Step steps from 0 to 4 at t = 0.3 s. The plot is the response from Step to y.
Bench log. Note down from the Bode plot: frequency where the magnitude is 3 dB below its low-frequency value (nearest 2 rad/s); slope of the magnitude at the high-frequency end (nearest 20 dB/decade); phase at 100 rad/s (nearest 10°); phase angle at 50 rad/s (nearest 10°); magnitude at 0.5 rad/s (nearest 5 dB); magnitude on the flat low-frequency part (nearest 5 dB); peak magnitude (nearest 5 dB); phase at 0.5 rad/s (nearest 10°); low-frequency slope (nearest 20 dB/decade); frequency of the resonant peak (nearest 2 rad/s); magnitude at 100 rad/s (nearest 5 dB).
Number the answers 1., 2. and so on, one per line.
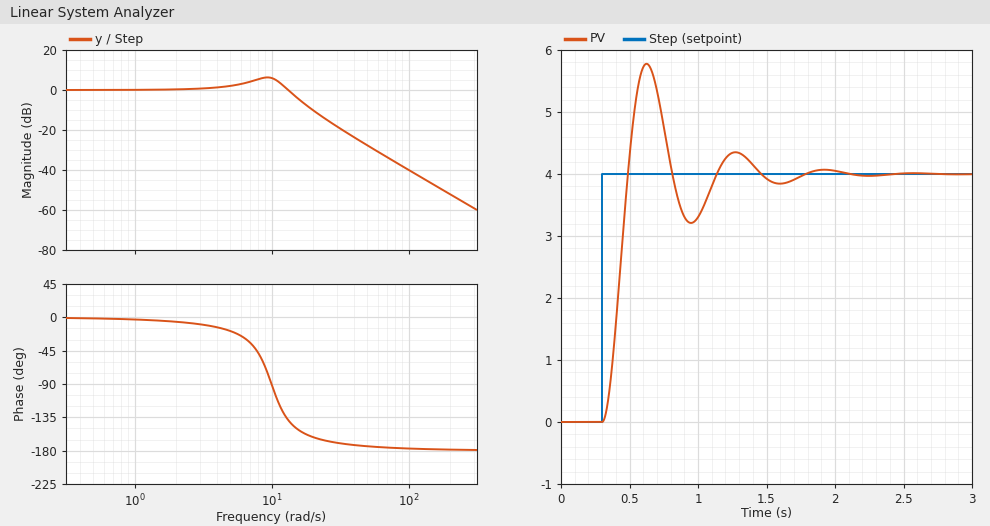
1. 14 rad/s
2. -40 dB/decade
3. -180°
4. -170°
5. 0 dB
6. 0 dB
7. 5 dB
8. 0°
9. 0 dB/decade
10. 10 rad/s
11. -40 dB
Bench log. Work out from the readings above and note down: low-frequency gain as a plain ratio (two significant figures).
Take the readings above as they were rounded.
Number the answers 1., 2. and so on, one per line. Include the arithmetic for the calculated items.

1. 10^(0 / 20) = 1.0
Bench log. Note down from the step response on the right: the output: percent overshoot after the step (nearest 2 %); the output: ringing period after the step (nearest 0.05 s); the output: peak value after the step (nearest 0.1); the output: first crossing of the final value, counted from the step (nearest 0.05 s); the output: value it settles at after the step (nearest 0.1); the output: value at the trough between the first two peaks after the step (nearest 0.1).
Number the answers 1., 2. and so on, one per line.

1. 44 %
2. 0.65 s
3. 5.8
4. 0.20 s
5. 4.0
6. 3.2
